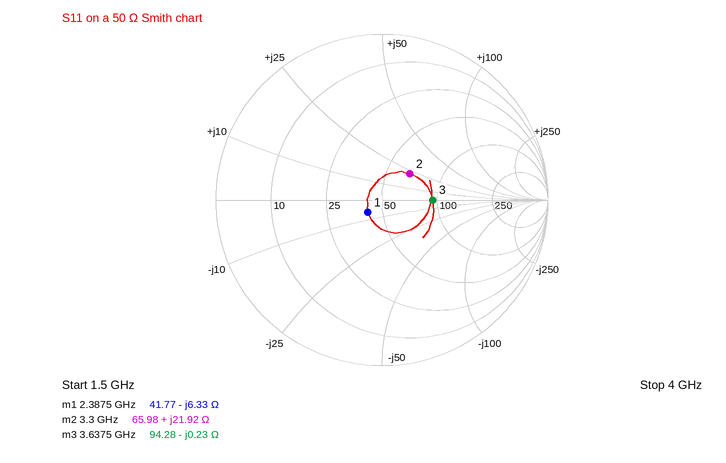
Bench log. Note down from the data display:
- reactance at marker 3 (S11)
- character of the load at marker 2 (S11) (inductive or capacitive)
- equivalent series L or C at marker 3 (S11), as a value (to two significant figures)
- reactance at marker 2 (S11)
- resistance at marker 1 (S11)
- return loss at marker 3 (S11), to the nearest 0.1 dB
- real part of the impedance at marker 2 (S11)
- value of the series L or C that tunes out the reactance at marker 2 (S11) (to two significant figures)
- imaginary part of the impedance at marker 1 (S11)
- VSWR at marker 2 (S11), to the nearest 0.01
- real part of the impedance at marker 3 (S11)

-0.23 Ω
inductive
190 pF
+21.92 Ω
41.77 Ω
10.3 dB
65.98 Ω
2.2 pF
-6.33 Ω
1.60
94.28 Ω
